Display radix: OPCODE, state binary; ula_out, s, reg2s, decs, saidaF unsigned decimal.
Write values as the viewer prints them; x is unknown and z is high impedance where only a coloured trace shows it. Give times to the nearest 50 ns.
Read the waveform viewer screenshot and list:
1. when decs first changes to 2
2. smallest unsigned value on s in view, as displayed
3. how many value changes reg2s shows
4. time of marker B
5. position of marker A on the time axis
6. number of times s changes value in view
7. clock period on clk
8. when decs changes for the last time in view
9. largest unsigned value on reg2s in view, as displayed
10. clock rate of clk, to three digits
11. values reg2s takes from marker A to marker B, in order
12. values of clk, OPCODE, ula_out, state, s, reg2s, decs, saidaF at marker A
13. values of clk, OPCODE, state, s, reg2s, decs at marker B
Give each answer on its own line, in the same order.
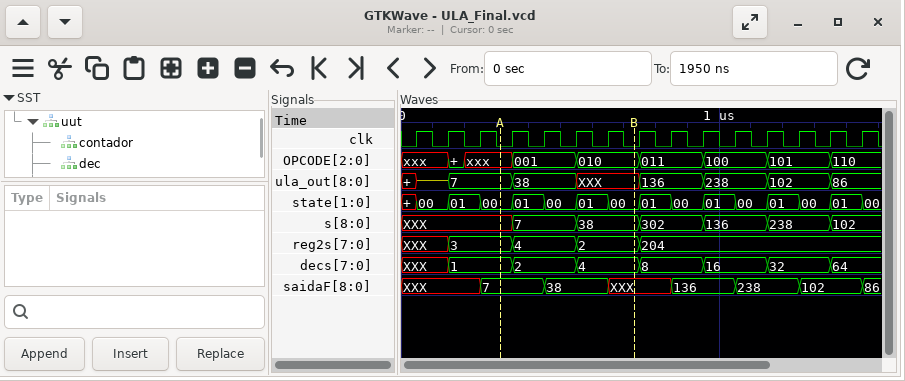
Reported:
350 ns
7
4
750 ns
300 ns
6
100 ns
1350 ns
204
10.0 MHz
3, 4, 2
clk=0, OPCODE=xxx, ula_out=7, state=00, s=XXX, reg2s=3, decs=1, saidaF=7
clk=0, OPCODE=010, state=00, s=38, reg2s=2, decs=4
